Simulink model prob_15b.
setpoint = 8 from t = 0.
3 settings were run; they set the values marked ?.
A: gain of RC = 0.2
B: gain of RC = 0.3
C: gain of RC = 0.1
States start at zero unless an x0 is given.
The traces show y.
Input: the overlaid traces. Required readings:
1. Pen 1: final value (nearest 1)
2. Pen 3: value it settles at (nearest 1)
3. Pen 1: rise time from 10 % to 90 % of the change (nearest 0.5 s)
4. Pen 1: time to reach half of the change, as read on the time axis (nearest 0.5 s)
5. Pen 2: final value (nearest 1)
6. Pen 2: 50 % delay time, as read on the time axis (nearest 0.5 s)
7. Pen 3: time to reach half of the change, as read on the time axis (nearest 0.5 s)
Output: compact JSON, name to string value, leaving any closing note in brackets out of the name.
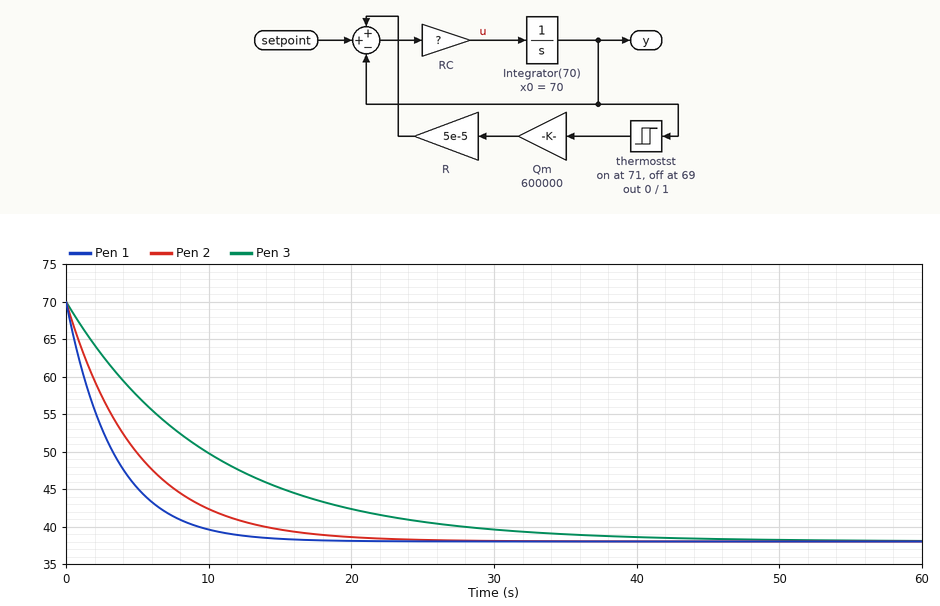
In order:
{"Pen 1: final value": "38", "Pen 3: value it settles at": "38", "Pen 1: rise time from 10 % to 90 % of the change": "7.5 s", "Pen 1: time to reach half of the change, as read on the time axis": "2.5 s", "Pen 2: final value": "38", "Pen 2: 50 % delay time, as read on the time axis": "3.5 s", "Pen 3: time to reach half of the change, as read on the time axis": "7.0 s"}
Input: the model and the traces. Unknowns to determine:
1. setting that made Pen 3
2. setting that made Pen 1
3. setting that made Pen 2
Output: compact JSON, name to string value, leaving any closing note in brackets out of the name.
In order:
{"setting that made Pen 3": "C", "setting that made Pen 1": "B", "setting that made Pen 2": "A"}
